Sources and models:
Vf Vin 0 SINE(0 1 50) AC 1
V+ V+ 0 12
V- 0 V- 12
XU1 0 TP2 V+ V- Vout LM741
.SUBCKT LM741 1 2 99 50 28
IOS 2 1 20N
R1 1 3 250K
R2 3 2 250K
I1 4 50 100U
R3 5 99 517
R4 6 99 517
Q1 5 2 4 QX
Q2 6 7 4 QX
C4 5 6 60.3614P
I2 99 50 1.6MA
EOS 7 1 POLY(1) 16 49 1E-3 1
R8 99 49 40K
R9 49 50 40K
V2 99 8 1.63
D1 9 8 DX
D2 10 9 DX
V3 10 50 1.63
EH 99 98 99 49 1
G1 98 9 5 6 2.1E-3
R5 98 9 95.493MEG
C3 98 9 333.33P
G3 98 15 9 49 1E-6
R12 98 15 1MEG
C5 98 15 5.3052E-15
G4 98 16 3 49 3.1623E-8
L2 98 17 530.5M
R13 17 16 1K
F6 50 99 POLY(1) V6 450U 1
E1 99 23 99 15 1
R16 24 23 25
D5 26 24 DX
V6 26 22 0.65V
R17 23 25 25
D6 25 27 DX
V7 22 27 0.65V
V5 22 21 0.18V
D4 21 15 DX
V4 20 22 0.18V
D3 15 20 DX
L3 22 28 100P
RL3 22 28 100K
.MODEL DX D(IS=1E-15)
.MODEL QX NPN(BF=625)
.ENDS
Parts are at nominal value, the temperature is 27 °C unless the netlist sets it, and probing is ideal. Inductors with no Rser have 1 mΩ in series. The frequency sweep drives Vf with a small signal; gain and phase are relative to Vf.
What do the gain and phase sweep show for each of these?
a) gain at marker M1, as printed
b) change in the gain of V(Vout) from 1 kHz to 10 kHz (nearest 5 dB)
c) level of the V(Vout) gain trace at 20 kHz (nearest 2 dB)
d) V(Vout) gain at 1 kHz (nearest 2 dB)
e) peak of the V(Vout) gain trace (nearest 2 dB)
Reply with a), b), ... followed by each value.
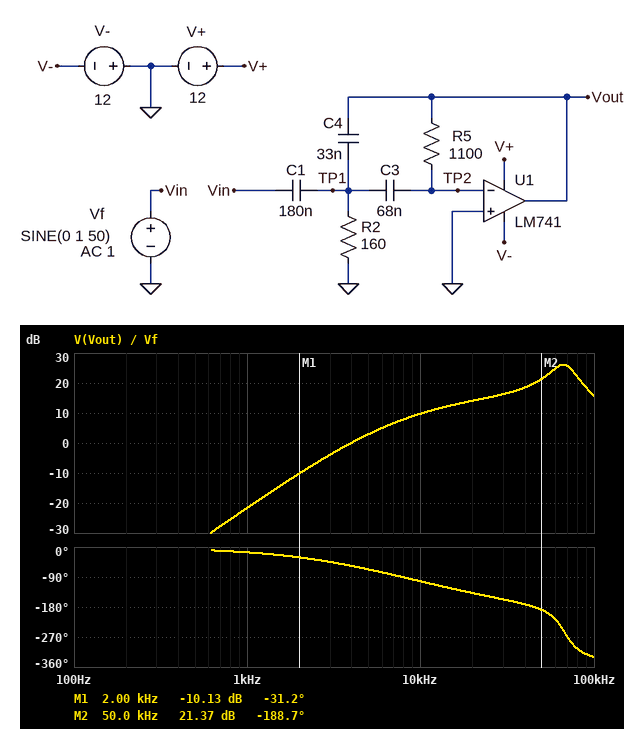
a) -10.13 dB
b) 30 dB
c) 14 dB
d) -22 dB
e) 26 dB
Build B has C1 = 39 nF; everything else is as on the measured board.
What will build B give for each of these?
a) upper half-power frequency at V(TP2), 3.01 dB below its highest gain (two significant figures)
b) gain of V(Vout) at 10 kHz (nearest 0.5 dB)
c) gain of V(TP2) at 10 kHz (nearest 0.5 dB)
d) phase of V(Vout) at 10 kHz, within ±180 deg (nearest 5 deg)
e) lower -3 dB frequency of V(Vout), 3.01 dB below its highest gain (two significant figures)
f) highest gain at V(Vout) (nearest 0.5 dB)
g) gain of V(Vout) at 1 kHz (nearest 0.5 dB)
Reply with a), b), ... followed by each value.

a) 210 kHz
b) 2.0 dB
c) -36.0 dB
d) -115 deg
e) 120 kHz
f) 14.5 dB
g) -34.5 dB
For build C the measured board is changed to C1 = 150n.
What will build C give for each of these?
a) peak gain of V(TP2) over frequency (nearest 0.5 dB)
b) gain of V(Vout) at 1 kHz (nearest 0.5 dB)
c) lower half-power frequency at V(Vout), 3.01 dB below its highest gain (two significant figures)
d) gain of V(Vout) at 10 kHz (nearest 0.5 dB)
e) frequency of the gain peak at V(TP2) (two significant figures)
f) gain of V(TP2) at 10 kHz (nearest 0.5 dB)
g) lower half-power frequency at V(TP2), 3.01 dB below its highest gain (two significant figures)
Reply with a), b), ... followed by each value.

a) 10.0 dB
b) -23.0 dB
c) 60 kHz
d) 9.0 dB
e) 77 kHz
f) -28.5 dB
g) 66 kHz
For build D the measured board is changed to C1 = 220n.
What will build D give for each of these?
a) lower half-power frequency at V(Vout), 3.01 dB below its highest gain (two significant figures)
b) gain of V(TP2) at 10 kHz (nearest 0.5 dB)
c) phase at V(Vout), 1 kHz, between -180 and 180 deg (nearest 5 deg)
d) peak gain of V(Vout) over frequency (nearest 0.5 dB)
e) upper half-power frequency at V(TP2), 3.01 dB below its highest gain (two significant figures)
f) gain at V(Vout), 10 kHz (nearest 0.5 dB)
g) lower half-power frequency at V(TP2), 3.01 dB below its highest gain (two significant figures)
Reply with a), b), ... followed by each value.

a) 51 kHz
b) -27.5 dB
c) -20 deg
d) 28.5 dB
e) 74 kHz
f) 10.5 dB
g) 54 kHz
